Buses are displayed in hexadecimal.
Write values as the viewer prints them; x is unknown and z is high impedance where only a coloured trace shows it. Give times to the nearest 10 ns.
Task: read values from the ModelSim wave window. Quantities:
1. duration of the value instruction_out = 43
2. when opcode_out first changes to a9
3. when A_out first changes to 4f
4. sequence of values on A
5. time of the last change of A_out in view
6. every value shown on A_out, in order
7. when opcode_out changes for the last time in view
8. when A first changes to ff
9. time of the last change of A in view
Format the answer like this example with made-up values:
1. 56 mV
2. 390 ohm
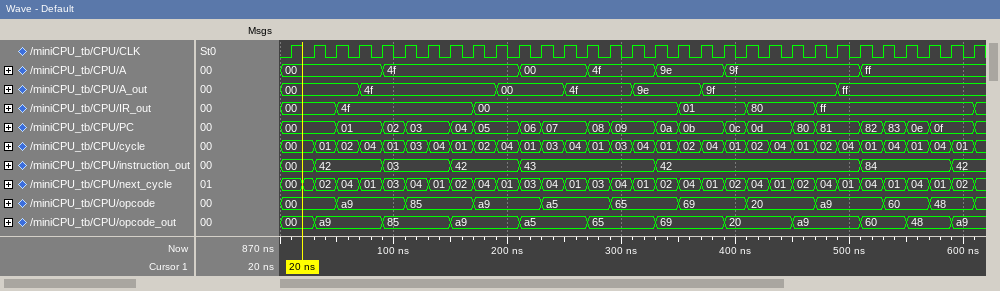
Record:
1. 120 ns
2. 30 ns
3. 70 ns
4. 00, 4f, 00, 4f, 9e, 9f, ff
5. 490 ns
6. 00, 4f, 00, 4f, 9e, 9f, ff
7. 590 ns
8. 510 ns
9. 510 ns
